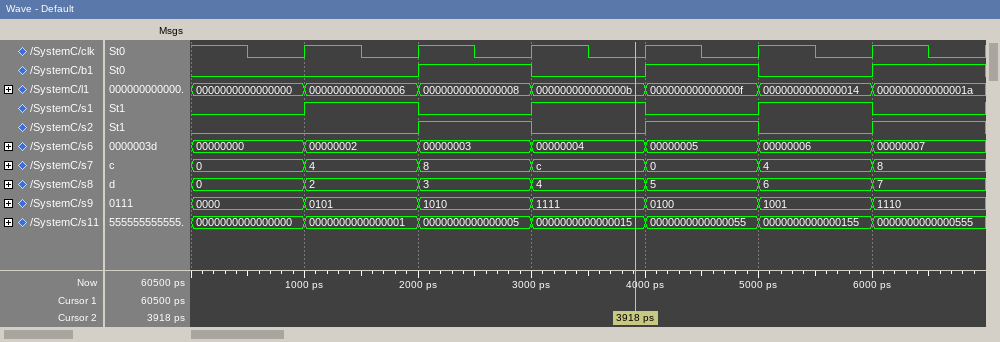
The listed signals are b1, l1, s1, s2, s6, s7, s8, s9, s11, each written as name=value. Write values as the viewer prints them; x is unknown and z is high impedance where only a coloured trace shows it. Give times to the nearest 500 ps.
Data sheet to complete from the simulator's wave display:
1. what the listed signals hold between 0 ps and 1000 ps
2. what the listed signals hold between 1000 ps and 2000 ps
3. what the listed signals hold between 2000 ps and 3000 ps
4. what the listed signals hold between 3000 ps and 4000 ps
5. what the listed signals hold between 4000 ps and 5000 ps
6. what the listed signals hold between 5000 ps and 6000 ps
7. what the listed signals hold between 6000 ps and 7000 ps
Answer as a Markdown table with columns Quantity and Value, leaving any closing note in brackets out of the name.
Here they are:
| Quantity | Value |
|---|---|
| what the listed signals hold between 0 ps and 1000 ps | b1=0, l1=0000000000000000, s1=0, s2=0, s6=00000000, s7=0, s8=0, s9=0000, s11=0000000000000000 |
| what the listed signals hold between 1000 ps and 2000 ps | b1=0, l1=0000000000000006, s1=1, s2=0, s6=00000002, s7=4, s8=2, s9=0101, s11=0000000000000001 |
| what the listed signals hold between 2000 ps and 3000 ps | b1=1, l1=0000000000000008, s1=0, s2=1, s6=00000003, s7=8, s8=3, s9=1010, s11=0000000000000005 |
| what the listed signals hold between 3000 ps and 4000 ps | b1=0, l1=000000000000000b, s1=1, s2=0, s6=00000004, s7=c, s8=4, s9=1111, s11=0000000000000015 |
| what the listed signals hold between 4000 ps and 5000 ps | b1=1, l1=000000000000000f, s1=0, s2=1, s6=00000005, s7=0, s8=5, s9=0100, s11=0000000000000055 |
| what the listed signals hold between 5000 ps and 6000 ps | b1=0, l1=0000000000000014, s1=1, s2=0, s6=00000006, s7=4, s8=6, s9=1001, s11=0000000000000155 |
| what the listed signals hold between 6000 ps and 7000 ps | b1=1, l1=000000000000001a, s1=0, s2=1, s6=00000007, s7=8, s8=7, s9=1110, s11=0000000000000555 |
